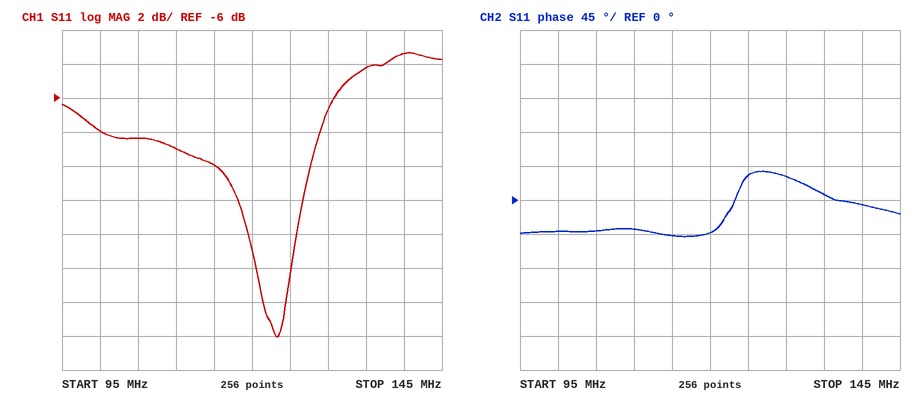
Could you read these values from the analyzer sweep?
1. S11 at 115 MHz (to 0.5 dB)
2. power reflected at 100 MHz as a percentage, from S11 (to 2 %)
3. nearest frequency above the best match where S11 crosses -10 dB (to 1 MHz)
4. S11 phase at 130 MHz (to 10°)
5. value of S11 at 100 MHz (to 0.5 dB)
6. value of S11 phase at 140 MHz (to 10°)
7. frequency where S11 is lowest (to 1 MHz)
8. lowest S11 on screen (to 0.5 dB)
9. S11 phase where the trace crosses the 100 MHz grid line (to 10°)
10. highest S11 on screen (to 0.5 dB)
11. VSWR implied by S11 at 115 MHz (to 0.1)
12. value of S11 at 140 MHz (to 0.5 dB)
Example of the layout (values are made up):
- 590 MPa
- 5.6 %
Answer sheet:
- -10.0 dB
- 16 %
- 128 MHz
- 30°
- -8.0 dB
- -10°
- 123 MHz
- -20.0 dB
- -40°
- -3.5 dB
- 1.9
- -3.5 dB
